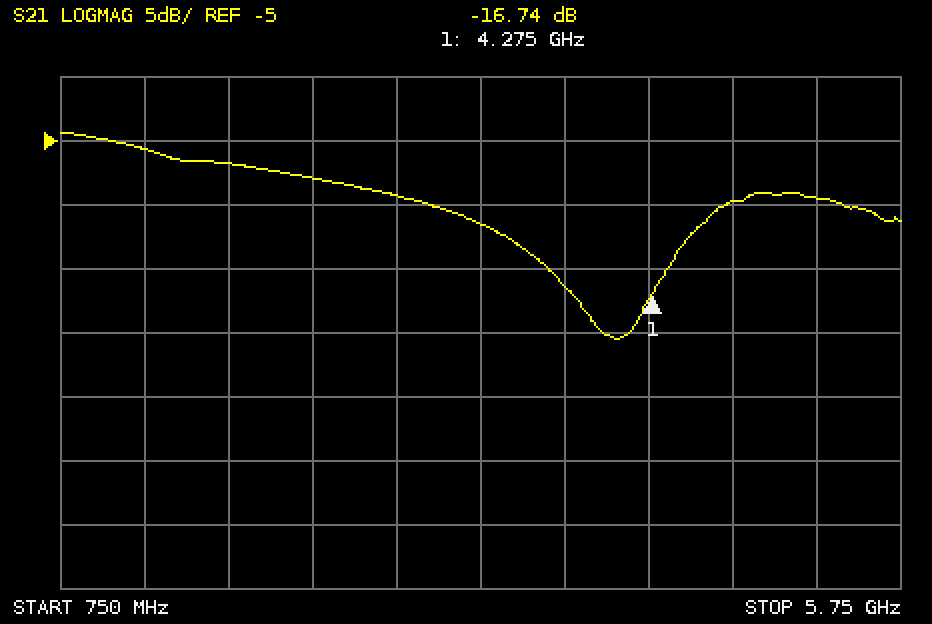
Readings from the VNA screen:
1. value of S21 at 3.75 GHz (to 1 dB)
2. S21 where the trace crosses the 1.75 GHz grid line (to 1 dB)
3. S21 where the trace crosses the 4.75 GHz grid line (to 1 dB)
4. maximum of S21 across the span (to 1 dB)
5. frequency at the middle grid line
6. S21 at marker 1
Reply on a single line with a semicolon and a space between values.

-16 dB; -7 dB; -10 dB; -4 dB; 3.25 GHz; -16.74 dB
